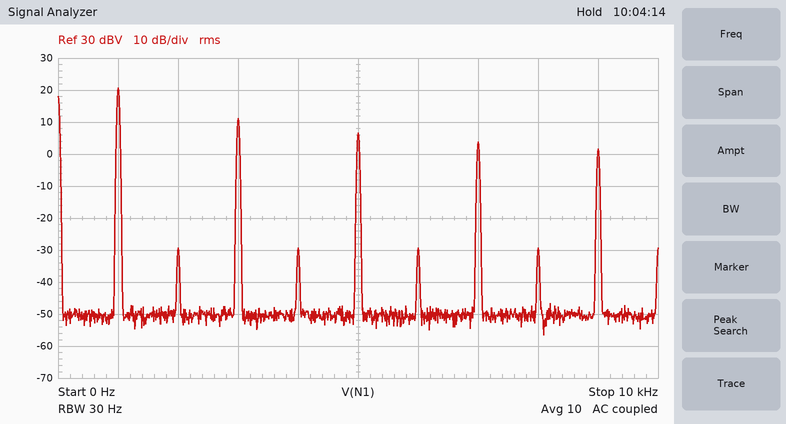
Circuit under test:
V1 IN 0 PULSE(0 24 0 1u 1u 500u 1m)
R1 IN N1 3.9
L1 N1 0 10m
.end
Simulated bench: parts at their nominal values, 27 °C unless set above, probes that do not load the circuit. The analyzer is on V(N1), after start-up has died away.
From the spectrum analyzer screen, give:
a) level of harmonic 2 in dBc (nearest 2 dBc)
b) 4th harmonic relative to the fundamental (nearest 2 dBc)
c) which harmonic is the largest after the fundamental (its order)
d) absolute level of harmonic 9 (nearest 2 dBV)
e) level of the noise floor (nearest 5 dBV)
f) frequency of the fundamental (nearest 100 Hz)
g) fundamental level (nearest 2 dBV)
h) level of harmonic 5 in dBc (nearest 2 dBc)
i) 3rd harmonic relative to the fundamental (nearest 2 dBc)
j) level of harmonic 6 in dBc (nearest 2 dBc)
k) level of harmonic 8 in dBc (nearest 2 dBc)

-50 dBc
-50 dBc
3
2 dBV
-50 dBV
1.0 kHz
20 dBV
-14 dBc
-10 dBc
-50 dBc
-50 dBc
